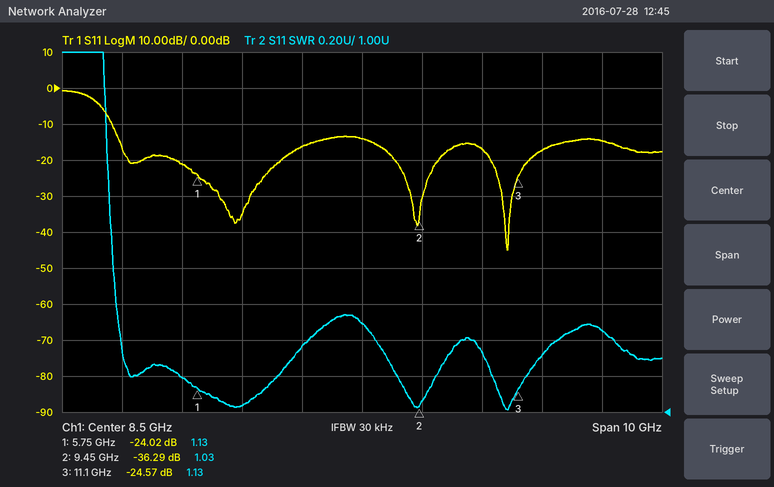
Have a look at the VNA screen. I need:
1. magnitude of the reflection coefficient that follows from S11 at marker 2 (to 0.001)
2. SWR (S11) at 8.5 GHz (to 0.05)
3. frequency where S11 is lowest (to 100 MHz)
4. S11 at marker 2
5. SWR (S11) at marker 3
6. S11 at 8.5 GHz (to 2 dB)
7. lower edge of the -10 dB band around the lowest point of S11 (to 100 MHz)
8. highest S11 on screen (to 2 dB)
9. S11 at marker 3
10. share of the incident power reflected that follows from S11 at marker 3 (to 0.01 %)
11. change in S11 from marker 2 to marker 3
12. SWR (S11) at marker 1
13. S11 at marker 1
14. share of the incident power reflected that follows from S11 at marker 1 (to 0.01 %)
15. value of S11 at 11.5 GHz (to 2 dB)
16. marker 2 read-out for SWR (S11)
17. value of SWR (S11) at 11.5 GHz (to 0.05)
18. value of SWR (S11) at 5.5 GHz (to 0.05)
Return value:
0.015
1.50
10.9 GHz
-36.29 dB
1.13
-14 dB
4.3 GHz
0 dB
-24.57 dB
0.35 %
11.72 dB
1.13
-24.02 dB
0.40 %
-18 dB
1.03
1.30
1.20
